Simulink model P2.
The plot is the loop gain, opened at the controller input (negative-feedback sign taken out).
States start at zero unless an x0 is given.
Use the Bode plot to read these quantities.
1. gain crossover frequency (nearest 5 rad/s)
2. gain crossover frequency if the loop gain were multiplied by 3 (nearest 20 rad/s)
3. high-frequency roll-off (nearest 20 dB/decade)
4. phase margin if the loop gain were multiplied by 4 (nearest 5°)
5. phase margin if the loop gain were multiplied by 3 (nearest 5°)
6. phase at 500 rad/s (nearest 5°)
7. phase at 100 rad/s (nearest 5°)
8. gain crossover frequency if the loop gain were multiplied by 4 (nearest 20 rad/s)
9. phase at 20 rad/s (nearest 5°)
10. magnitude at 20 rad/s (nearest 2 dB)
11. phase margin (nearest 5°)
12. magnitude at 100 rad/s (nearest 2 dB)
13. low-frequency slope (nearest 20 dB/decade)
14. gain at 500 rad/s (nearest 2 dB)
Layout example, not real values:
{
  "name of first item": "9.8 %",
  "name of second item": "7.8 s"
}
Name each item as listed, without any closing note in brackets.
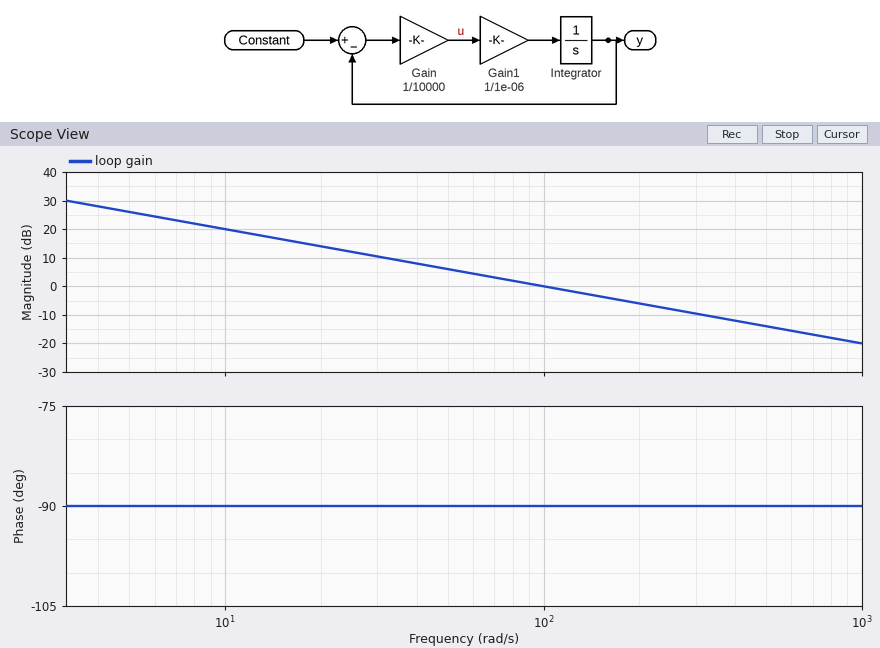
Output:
{
  "gain crossover frequency": "100 rad/s",
  "gain crossover frequency if the loop gain were multiplied by 3": "300 rad/s",
  "high-frequency roll-off": "-20 dB/decade",
  "phase margin if the loop gain were multiplied by 4": "90°",
  "phase margin if the loop gain were multiplied by 3": "90°",
  "phase at 500 rad/s": "-90°",
  "phase at 100 rad/s": "-90°",
  "gain crossover frequency if the loop gain were multiplied by 4": "400 rad/s",
  "phase at 20 rad/s": "-90°",
  "magnitude at 20 rad/s": "14 dB",
  "phase margin": "90°",
  "magnitude at 100 rad/s": "0 dB",
  "low-frequency slope": "-20 dB/decade",
  "gain at 500 rad/s": "-14 dB"
}
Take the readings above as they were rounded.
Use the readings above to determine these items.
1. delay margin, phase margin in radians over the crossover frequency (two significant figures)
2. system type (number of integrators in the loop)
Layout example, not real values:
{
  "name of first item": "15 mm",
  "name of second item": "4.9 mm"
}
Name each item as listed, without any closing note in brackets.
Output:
{
  "delay margin, phase margin in radians over the crossover frequency": "0.016 s",
  "system type": "1"
}
